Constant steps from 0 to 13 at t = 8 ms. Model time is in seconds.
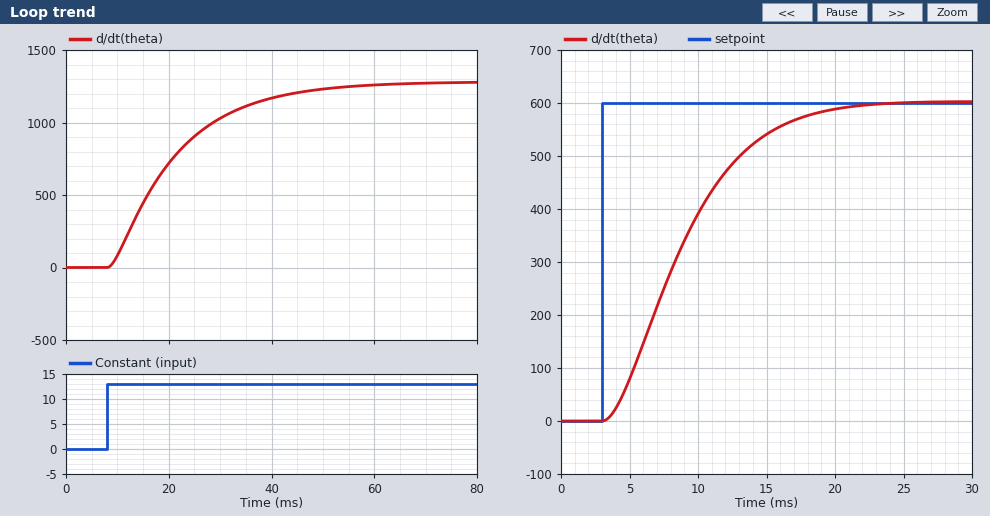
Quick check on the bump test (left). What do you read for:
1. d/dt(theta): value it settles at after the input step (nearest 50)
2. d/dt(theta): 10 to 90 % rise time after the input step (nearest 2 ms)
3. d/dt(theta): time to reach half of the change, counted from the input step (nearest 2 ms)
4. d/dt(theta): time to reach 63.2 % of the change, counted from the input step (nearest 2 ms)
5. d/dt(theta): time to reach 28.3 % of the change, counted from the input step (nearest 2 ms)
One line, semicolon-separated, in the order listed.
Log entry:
1300; 28 ms; 10 ms; 14 ms; 6 ms
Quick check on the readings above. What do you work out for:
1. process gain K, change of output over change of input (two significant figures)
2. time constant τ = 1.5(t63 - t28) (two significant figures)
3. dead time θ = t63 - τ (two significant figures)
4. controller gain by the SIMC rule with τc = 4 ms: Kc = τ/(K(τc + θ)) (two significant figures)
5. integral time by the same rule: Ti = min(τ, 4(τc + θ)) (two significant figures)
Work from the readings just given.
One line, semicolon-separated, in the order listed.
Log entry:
100; 12 ms; 2.0 ms; 0.020; 12 ms
